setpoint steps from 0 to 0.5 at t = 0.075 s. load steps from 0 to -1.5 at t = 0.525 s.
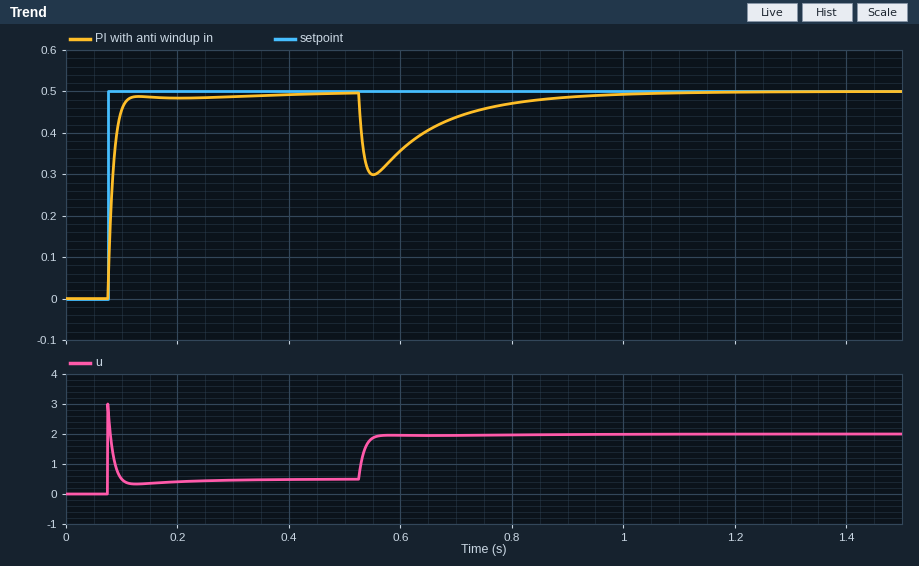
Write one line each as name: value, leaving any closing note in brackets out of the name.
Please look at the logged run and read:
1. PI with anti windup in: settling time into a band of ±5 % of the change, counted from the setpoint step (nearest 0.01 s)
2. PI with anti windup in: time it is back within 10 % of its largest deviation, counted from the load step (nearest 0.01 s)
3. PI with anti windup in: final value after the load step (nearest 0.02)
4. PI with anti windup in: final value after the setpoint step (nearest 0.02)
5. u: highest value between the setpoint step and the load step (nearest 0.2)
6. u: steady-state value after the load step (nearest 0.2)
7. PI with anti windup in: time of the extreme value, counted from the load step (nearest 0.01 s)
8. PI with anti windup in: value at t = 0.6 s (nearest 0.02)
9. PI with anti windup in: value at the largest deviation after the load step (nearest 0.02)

PI with anti windup in: settling time into a band of ±5 % of the change, counted from the setpoint step: 0.03 s
PI with anti windup in: time it is back within 10 % of its largest deviation, counted from the load step: 0.33 s
PI with anti windup in: final value after the load step: 0.50
PI with anti windup in: final value after the setpoint step: 0.50
u: highest value between the setpoint step and the load step: 3.0
u: steady-state value after the load step: 2.0
PI with anti windup in: time of the extreme value, counted from the load step: 0.03 s
PI with anti windup in: value at t = 0.6 s: 0.36
PI with anti windup in: value at the largest deviation after the load step: 0.30
